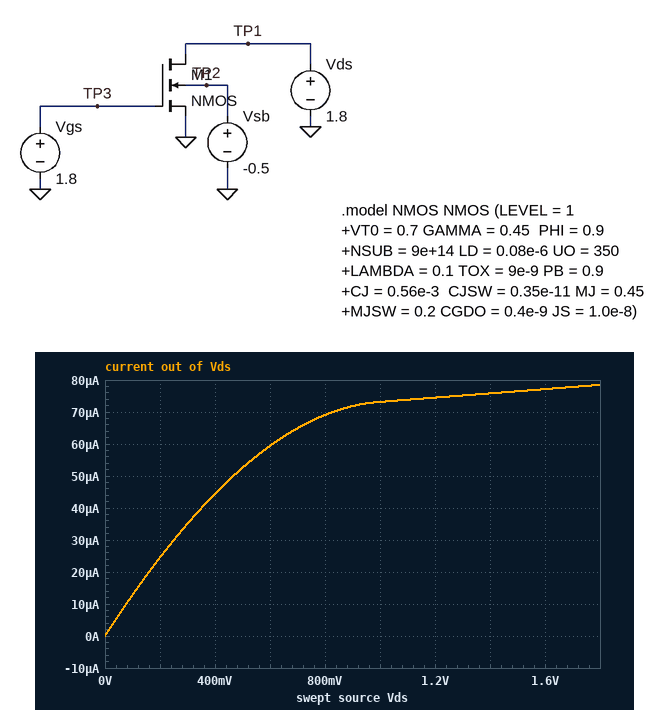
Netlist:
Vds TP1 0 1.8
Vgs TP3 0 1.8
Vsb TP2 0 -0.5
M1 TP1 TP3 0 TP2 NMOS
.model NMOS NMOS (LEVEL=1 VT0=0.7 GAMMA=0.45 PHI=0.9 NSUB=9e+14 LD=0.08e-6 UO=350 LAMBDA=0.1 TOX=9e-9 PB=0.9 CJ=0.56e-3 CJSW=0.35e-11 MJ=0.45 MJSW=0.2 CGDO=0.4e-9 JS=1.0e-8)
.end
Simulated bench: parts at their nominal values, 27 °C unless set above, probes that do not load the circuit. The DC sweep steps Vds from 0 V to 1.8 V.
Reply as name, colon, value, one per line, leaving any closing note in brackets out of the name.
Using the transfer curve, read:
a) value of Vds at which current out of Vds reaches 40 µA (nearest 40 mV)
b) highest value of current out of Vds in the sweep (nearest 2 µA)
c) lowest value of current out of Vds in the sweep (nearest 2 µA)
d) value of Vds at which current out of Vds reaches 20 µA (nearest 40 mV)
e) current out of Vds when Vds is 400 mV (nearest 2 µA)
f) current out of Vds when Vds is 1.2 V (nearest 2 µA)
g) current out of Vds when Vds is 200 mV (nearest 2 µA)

value of Vds at which current out of Vds reaches 40 µA: 360 mV
highest value of current out of Vds in the sweep: 78 µA
lowest value of current out of Vds in the sweep: 0 A
value of Vds at which current out of Vds reaches 20 µA: 160 mV
current out of Vds when Vds is 400 mV: 44 µA
current out of Vds when Vds is 1.2 V: 74 µA
current out of Vds when Vds is 200 mV: 24 µA
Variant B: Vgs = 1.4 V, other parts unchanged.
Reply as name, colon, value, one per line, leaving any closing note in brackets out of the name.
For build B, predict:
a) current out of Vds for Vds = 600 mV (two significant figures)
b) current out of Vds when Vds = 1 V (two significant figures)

current out of Vds for Vds = 600 mV: 25 µA
current out of Vds when Vds = 1 V: 26 µA
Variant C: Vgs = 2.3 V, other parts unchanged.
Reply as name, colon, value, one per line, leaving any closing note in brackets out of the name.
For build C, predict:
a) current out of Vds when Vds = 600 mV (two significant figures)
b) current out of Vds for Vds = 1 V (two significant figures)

current out of Vds when Vds = 600 mV: 100 µA
current out of Vds for Vds = 1 V: 150 µA
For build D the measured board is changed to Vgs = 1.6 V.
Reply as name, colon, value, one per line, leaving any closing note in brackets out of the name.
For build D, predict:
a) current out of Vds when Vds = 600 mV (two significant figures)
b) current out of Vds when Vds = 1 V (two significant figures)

current out of Vds when Vds = 600 mV: 42 µA
current out of Vds when Vds = 1 V: 47 µA
